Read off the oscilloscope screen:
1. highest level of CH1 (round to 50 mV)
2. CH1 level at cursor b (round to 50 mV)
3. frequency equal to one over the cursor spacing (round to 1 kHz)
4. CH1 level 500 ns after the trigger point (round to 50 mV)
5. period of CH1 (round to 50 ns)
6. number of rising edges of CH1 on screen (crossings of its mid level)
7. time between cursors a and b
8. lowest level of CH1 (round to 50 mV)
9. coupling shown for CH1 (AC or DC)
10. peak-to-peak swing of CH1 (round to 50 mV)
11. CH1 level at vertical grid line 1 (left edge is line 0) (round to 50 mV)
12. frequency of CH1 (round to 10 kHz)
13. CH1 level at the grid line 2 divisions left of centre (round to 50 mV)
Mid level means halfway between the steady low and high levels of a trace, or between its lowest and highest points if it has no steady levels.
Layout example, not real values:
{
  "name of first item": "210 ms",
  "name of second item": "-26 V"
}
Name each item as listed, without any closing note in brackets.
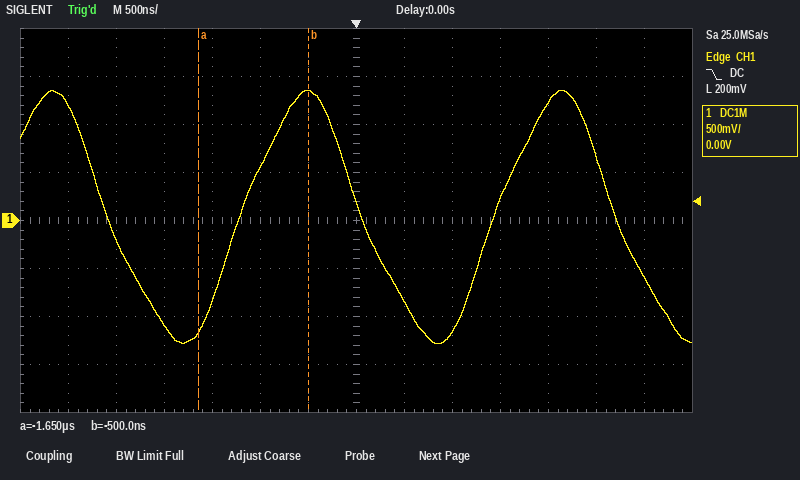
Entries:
{
  "highest level of CH1": "1.35 V",
  "CH1 level at cursor b": "1.35 V",
  "frequency equal to one over the cursor spacing": "870 kHz",
  "CH1 level 500 ns after the trigger point": "-850 mV",
  "period of CH1": "2.65 µs",
  "number of rising edges of CH1 on screen": "2",
  "time between cursors a and b": "1.15 µs",
  "lowest level of CH1": "-1.30 V",
  "coupling shown for CH1": "DC",
  "peak-to-peak swing of CH1": "2.65 V",
  "CH1 level at vertical grid line 1 (left edge is line 0)": "1.20 V",
  "frequency of CH1": "380 kHz",
  "CH1 level at the grid line 2 divisions left of centre": "550 mV"
}
